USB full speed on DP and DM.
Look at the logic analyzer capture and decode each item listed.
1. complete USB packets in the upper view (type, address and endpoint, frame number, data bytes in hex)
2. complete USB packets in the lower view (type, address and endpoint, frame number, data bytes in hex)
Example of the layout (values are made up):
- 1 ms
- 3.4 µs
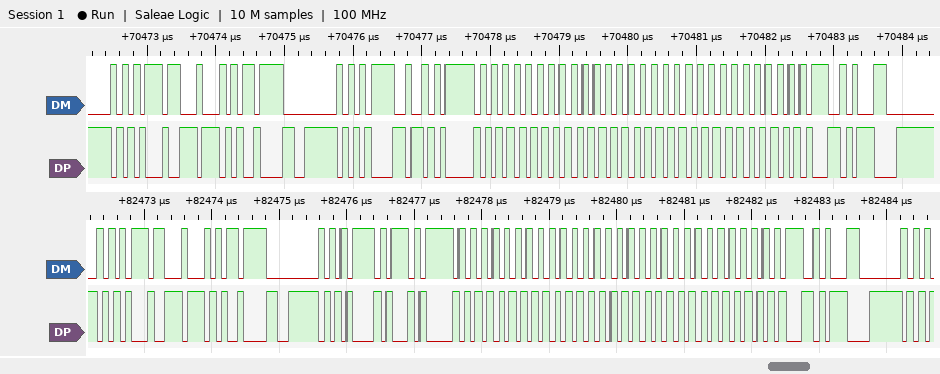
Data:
- IN ADDR 6 EP 2, DATA1 [ F0 00 00 00 00 00 00 00 ]
- IN ADDR 6 EP 2, DATA0 [ F0 00 00 00 00 00 00 00 ]
